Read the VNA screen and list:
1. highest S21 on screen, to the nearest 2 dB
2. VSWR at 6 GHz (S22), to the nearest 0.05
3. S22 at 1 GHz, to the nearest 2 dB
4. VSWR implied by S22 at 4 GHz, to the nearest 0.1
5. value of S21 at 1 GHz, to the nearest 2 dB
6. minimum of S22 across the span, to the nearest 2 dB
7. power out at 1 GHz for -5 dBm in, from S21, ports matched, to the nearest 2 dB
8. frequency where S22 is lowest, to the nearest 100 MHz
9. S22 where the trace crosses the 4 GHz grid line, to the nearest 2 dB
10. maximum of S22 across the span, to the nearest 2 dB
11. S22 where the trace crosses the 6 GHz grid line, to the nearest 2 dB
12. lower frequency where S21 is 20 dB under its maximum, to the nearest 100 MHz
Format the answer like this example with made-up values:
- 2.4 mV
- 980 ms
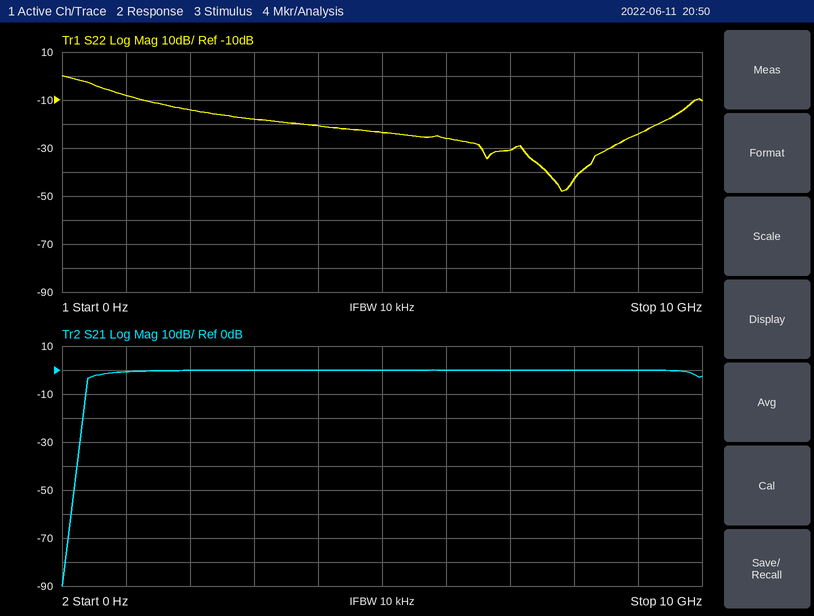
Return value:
- 0 dB
- 1.10
- -8 dB
- 1.2
- 0 dB
- -48 dB
- -6 dBm
- 7.8 GHz
- -20 dB
- 0 dB
- -26 dB
- 300 MHz
